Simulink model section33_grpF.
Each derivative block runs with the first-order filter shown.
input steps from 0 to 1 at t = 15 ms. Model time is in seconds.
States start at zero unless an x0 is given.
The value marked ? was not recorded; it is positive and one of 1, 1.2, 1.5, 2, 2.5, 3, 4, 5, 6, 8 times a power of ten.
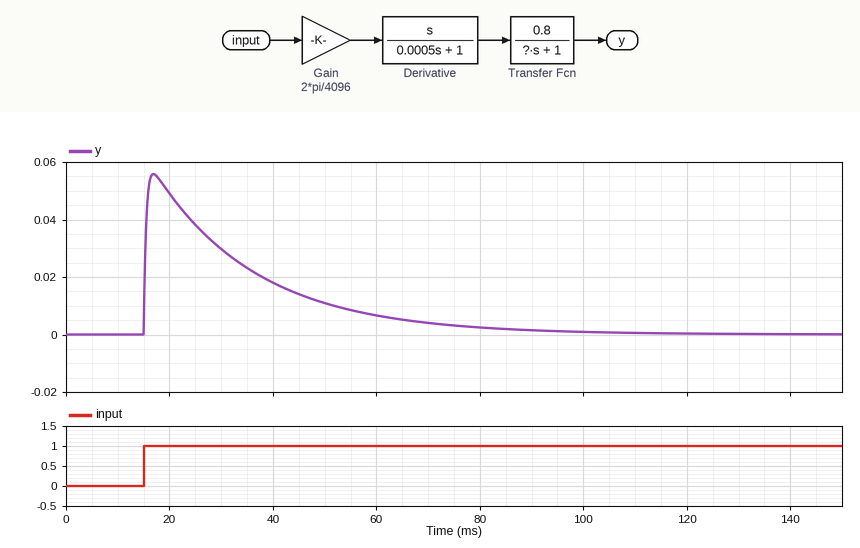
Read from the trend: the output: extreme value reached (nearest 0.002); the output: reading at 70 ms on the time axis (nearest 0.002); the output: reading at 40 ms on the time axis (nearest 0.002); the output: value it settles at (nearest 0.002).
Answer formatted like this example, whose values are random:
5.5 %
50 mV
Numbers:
0.056
0.004
0.018
0.000
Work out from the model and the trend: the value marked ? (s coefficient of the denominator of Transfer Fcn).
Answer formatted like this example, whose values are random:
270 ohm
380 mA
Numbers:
0.02
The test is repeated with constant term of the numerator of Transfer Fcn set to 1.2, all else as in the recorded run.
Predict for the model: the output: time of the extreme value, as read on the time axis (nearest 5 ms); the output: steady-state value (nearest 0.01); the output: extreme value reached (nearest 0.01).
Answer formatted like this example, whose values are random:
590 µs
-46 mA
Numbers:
15 ms
0.00
0.08
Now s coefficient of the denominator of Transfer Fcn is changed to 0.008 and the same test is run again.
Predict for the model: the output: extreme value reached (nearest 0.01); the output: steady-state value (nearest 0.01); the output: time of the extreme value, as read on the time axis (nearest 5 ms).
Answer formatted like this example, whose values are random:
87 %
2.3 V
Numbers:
0.13
0.00
15 ms
